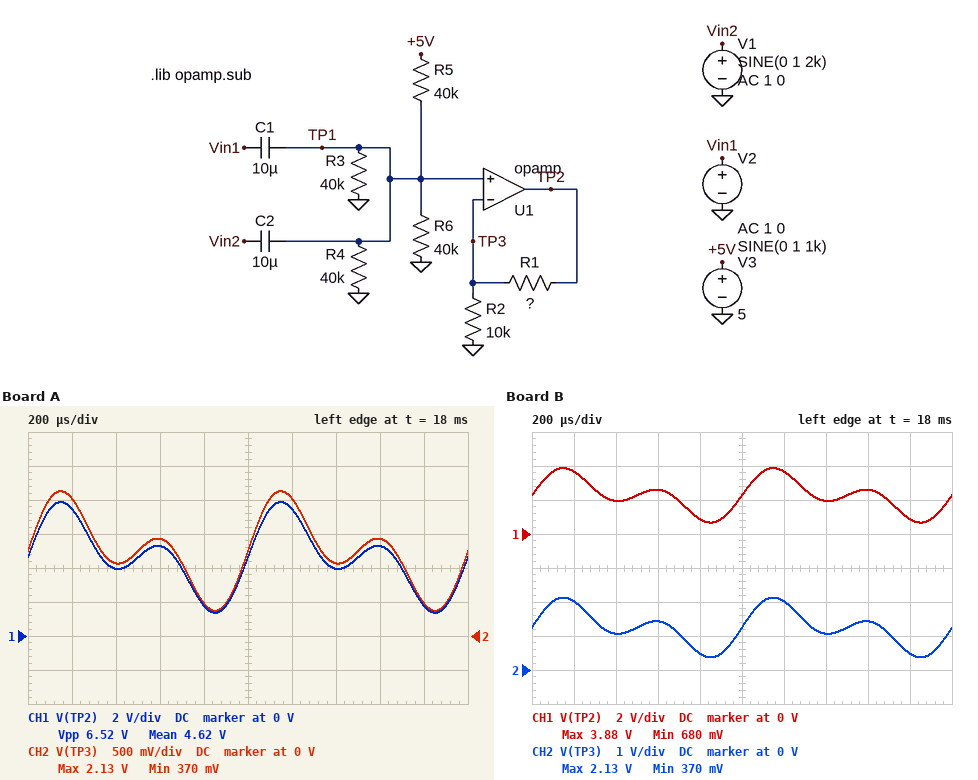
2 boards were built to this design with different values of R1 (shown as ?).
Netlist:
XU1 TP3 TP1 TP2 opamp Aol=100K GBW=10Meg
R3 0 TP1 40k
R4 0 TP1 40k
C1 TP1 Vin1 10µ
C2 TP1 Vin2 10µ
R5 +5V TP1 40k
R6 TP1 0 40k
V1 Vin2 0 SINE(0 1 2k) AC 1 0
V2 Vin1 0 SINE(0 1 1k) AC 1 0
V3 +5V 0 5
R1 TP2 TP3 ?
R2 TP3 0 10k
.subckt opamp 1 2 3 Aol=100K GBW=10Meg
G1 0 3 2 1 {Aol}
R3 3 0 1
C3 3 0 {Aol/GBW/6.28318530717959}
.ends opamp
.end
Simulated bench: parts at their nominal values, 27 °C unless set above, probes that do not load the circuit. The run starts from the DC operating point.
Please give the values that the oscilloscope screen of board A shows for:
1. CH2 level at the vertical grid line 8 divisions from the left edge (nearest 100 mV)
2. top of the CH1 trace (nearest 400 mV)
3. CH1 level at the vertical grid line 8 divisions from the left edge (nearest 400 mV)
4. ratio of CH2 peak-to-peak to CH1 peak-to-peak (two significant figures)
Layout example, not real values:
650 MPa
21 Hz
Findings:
1.4 V
8.0 V
5.2 V
0.27
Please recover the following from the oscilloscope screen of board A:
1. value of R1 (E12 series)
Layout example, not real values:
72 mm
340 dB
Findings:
27 kΩ
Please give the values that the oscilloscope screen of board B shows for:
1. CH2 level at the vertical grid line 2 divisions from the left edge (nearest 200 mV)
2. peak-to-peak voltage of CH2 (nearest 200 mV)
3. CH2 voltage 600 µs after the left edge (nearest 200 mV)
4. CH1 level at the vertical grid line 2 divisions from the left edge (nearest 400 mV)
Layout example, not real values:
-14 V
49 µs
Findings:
1.0 V
1.8 V
1.4 V
2.0 V
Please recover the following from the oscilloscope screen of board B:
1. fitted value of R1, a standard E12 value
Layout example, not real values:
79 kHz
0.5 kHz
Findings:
8.2 kΩ
